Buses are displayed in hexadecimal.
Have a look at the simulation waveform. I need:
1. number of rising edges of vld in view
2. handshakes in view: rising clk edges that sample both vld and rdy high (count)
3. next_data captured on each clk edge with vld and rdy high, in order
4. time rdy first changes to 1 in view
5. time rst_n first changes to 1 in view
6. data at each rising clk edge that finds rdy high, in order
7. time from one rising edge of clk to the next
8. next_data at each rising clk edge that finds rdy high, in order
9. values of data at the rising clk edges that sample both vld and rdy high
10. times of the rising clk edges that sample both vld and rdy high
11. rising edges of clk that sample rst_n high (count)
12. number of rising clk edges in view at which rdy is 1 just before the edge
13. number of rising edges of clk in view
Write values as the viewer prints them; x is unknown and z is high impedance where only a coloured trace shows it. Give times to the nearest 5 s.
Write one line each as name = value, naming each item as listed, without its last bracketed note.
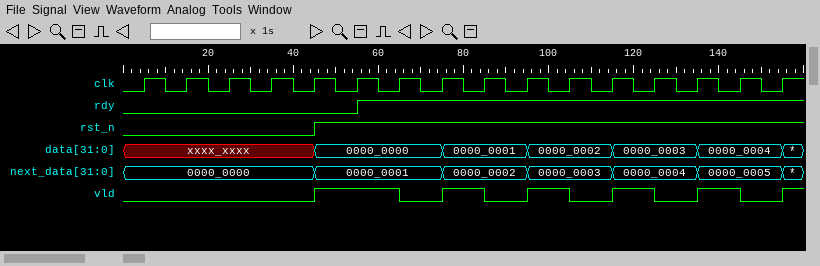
number of rising edges of vld in view = 6
handshakes in view: rising clk edges that sample both vld and rdy high = 5
next_data captured on each clk edge with vld and rdy high, in order = 0000_0001, 0000_0002, 0000_0003, 0000_0004, 0000_0005
time rdy first changes to 1 in view = 55 s
time rst_n first changes to 1 in view = 45 s
data at each rising clk edge that finds rdy high, in order = 0000_0000, 0000_0000, 0000_0001, 0000_0001, 0000_0002, 0000_0002, 0000_0003, 0000_0003, 0000_0004, 0000_0004
time from one rising edge of clk to the next = 10 s
next_data at each rising clk edge that finds rdy high, in order = 0000_0001, 0000_0001, 0000_0002, 0000_0002, 0000_0003, 0000_0003, 0000_0004, 0000_0004, 0000_0005, 0000_0005
values of data at the rising clk edges that sample both vld and rdy high = 0000_0000, 0000_0001, 0000_0002, 0000_0003, 0000_0004
times of the rising clk edges that sample both vld and rdy high = 65 s, 85 s, 105 s, 125 s, 145 s
rising edges of clk that sample rst_n high = 11
number of rising clk edges in view at which rdy is 1 just before the edge = 10
number of rising edges of clk in view = 16
